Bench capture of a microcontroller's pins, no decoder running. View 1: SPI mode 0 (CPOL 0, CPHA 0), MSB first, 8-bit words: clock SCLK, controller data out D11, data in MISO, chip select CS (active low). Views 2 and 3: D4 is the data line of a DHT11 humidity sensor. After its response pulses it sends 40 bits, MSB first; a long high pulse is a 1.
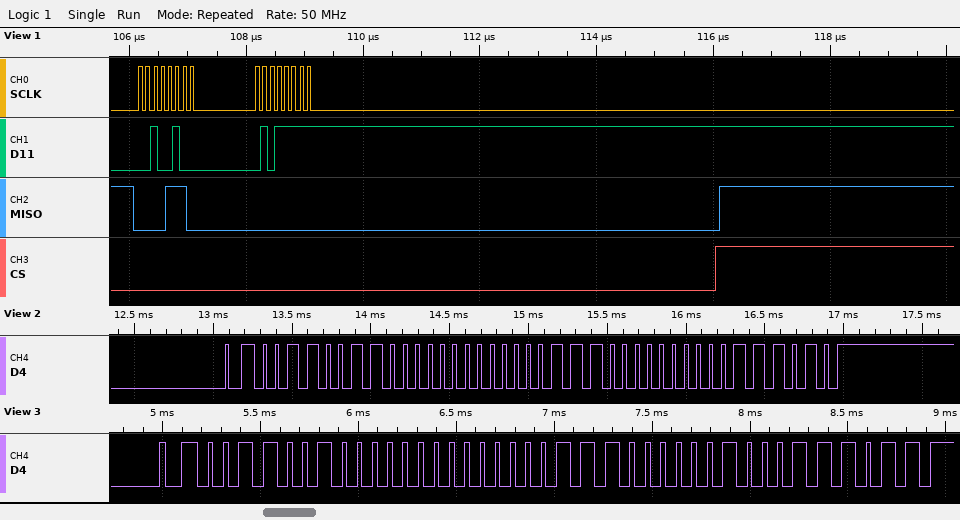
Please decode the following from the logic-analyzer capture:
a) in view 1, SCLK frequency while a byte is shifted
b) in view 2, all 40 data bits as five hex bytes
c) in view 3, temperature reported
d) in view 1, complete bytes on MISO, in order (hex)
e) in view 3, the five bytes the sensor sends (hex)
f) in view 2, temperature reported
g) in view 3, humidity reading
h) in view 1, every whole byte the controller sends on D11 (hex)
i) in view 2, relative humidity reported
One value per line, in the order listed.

8 MHz
33 00 07 00 3A
7.2 °C
0x0E 0x00
32 00 07 02 3B
7.0 °C
50 %
0x24 0x5F
51 %
